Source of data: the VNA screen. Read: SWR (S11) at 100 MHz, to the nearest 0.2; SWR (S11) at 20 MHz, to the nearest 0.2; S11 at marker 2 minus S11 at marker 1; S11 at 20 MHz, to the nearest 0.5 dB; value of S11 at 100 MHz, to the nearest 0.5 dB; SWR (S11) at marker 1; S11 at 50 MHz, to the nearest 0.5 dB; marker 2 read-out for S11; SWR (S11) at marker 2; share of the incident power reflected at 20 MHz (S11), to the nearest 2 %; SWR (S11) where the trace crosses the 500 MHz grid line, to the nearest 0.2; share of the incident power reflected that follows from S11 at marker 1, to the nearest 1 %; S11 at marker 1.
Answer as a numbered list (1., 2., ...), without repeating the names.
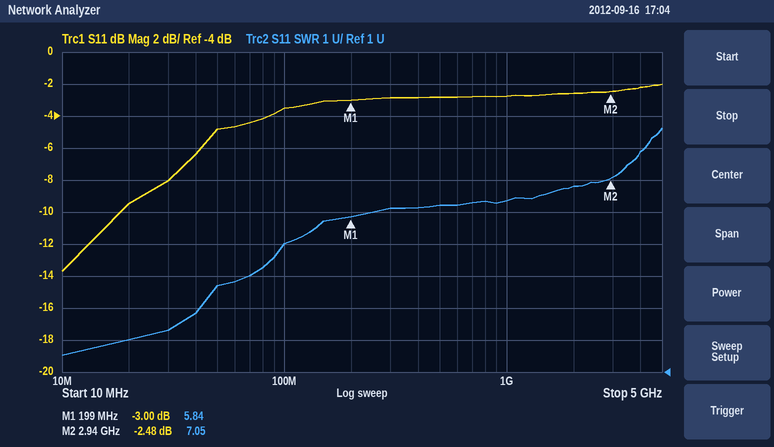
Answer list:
1. 5.0
2. 2.0
3. 0.52 dB
4. -9.5 dB
5. -3.5 dB
6. 5.84
7. -5.0 dB
8. -2.48 dB
9. 7.05
10. 12 %
11. 6.2
12. 50 %
13. -3.00 dB
